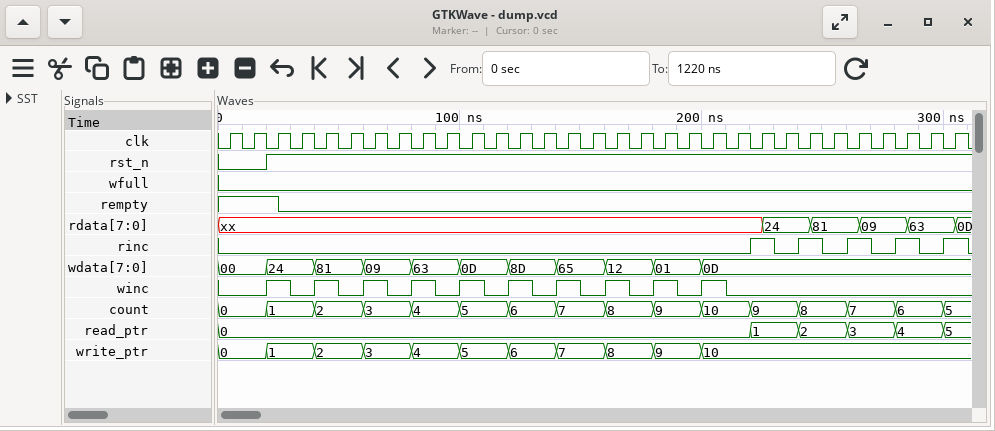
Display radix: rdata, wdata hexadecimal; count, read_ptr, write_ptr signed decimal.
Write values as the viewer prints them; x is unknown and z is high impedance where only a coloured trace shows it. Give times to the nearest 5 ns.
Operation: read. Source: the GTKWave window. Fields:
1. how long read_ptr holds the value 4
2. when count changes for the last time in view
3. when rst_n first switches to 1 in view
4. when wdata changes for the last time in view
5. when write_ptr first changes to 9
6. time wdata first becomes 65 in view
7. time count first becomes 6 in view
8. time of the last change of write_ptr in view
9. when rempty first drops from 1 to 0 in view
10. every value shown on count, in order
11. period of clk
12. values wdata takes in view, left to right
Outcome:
20 ns
300 ns
20 ns
200 ns
180 ns
140 ns
120 ns
200 ns
25 ns
0, 1, 2, 3, 4, 5, 6, 7, 8, 9, 10, 9, 8, 7, 6, 5
10 ns
00, 24, 81, 09, 63, 0D, 8D, 65, 12, 01, 0D
